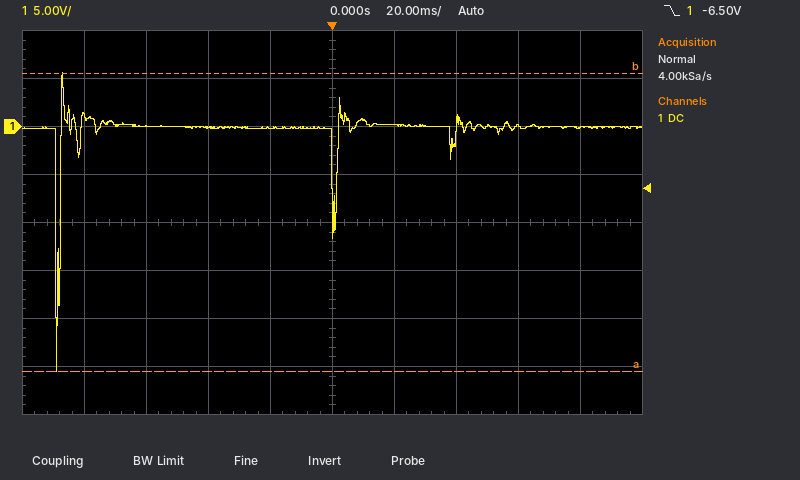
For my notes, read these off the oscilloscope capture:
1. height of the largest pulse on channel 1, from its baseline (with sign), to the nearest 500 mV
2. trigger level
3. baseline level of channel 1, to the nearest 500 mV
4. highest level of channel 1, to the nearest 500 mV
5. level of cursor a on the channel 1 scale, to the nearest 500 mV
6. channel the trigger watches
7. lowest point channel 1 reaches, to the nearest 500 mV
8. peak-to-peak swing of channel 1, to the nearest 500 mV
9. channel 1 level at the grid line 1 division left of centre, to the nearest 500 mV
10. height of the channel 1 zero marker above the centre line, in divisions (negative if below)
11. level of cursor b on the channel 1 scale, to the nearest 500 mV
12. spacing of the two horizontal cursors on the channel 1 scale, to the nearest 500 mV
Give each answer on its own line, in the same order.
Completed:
-25.5 V
-6.50 V
0.0 V
5.5 V
-25.5 V
channel 1
-25.5 V
31.0 V
0.0 V
+2.0 div
5.5 V
31.0 V
